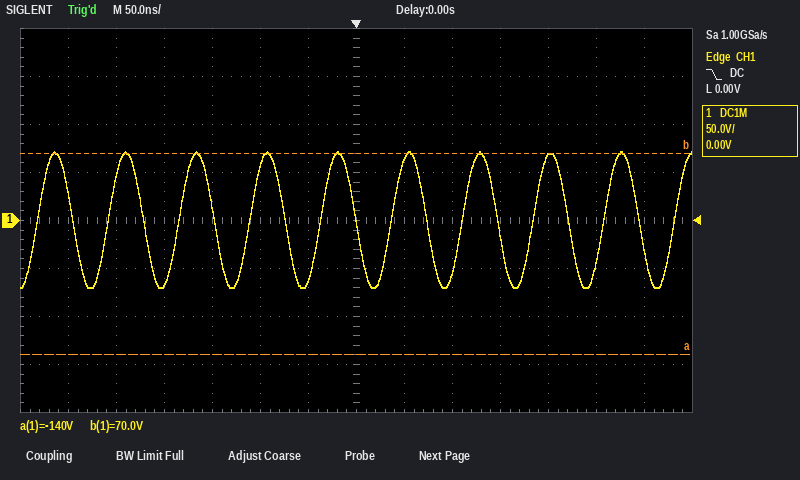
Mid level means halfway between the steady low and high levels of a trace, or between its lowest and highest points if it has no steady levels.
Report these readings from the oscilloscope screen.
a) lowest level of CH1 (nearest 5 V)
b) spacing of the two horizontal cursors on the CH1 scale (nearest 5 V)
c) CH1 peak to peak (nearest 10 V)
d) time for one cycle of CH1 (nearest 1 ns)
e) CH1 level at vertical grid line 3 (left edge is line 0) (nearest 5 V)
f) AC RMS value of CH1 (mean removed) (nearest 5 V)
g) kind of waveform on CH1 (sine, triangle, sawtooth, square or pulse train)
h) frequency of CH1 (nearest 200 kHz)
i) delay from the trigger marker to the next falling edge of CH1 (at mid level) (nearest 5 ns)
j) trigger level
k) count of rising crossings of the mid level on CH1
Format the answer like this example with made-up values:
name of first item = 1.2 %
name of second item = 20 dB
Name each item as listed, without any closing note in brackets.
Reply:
lowest level of CH1 = -70 V
spacing of the two horizontal cursors on the CH1 scale = 210 V
CH1 peak to peak = 140 V
time for one cycle of CH1 = 74 ns
CH1 level at vertical grid line 3 (left edge is line 0) = -65 V
AC RMS value of CH1 (mean removed) = 50 V
kind of waveform on CH1 = sine
frequency of CH1 = 13.6 MHz
delay from the trigger marker to the next falling edge of CH1 (at mid level) = 75 ns
trigger level = 0.00 V
count of rising crossings of the mid level on CH1 = 10
